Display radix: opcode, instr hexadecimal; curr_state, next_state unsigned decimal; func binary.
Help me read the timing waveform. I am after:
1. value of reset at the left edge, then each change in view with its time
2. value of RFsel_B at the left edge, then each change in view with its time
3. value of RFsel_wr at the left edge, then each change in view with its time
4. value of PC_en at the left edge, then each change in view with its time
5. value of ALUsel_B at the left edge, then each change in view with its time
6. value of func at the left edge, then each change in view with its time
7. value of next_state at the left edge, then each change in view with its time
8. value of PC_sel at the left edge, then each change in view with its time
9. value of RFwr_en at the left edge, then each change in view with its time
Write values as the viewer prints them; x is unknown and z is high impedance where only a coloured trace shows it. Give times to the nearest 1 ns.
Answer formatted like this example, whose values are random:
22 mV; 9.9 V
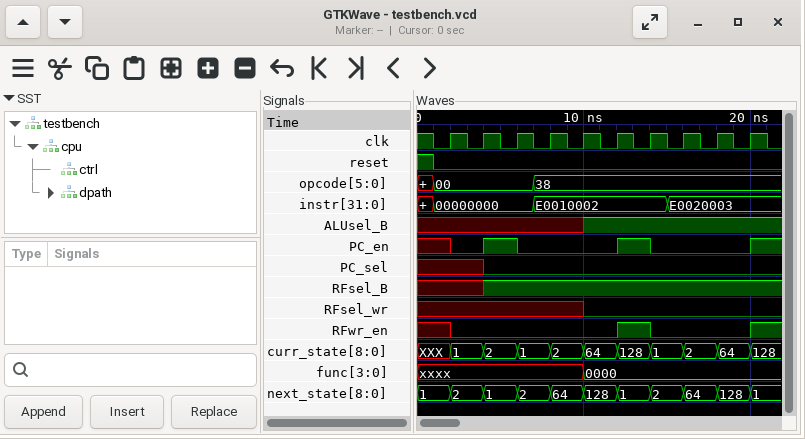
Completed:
1, 0 at 1 ns; x, 1 at 4 ns; x, 0 at 10 ns; x, 0 at 2 ns, 1 at 4 ns, 0 at 6 ns, 1 at 12 ns, 0 at 14 ns, 1 at 20 ns; x, 1 at 10 ns; xxxx, 0000 at 10 ns; 1, 2 at 2 ns, 1 at 4 ns, 2 at 6 ns, 64 at 8 ns, 128 at 10 ns, 1 at 12 ns, 2 at 14 ns, 64 at 16 ns, 128 at 18 ns, 1 at 20 ns; x, 0 at 4 ns; x, 0 at 2 ns, 1 at 12 ns, 0 at 14 ns, 1 at 20 ns
